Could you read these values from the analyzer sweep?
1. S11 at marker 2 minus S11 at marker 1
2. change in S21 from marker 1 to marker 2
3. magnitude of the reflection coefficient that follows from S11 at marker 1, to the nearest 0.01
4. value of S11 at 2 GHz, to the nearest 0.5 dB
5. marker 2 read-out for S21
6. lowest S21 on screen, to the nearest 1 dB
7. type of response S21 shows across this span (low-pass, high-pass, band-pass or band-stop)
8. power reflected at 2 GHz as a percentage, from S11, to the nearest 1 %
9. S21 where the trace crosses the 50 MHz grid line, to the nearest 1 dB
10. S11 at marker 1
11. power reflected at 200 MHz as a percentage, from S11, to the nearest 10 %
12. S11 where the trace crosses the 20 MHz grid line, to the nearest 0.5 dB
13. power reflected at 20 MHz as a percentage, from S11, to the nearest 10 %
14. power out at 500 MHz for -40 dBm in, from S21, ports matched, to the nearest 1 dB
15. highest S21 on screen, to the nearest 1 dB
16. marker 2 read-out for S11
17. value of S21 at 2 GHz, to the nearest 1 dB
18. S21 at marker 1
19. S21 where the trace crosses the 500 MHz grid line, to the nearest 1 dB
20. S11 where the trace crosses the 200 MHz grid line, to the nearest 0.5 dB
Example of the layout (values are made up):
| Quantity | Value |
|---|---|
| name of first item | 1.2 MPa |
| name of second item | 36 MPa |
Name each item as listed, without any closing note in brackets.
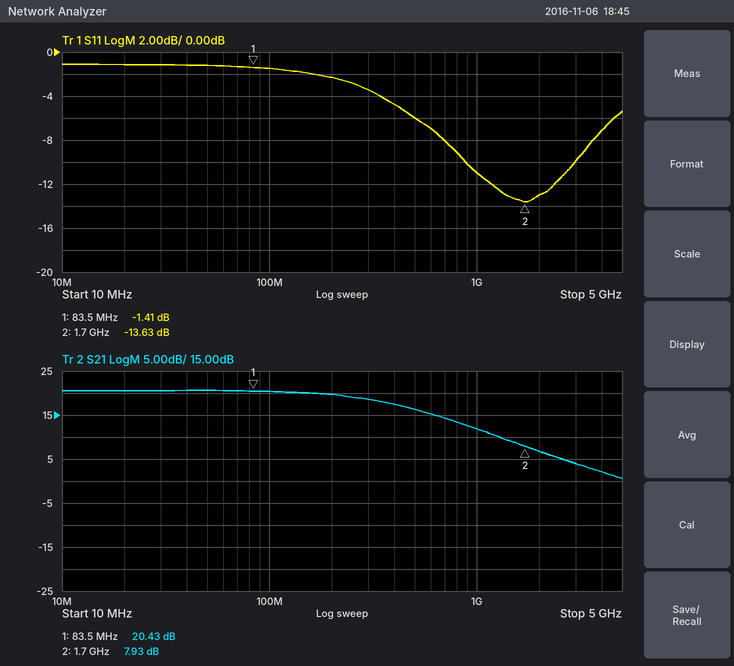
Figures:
| Quantity | Value |
|---|---|
| S11 at marker 2 minus S11 at marker 1 | -12.22 dB |
| change in S21 from marker 1 to marker 2 | -12.50 dB |
| magnitude of the reflection coefficient that follows from S11 at marker 1, to the nearest 0.01 | 0.85 |
| value of S11 at 2 GHz, to the nearest 0.5 dB | -13.0 dB |
| marker 2 read-out for S21 | 7.93 dB |
| lowest S21 on screen, to the nearest 1 dB | 1 dB |
| type of response S21 shows across this span | low-pass |
| power reflected at 2 GHz as a percentage, from S11, to the nearest 1 % | 5 % |
| S21 where the trace crosses the 50 MHz grid line, to the nearest 1 dB | 21 dB |
| S11 at marker 1 | -1.41 dB |
| power reflected at 200 MHz as a percentage, from S11, to the nearest 10 % | 60 % |
| S11 where the trace crosses the 20 MHz grid line, to the nearest 0.5 dB | -1.0 dB |
| power reflected at 20 MHz as a percentage, from S11, to the nearest 10 % | 80 % |
| power out at 500 MHz for -40 dBm in, from S21, ports matched, to the nearest 1 dB | -24 dBm |
| highest S21 on screen, to the nearest 1 dB | 21 dB |
| marker 2 read-out for S11 | -13.63 dB |
| value of S21 at 2 GHz, to the nearest 1 dB | 7 dB |
| S21 at marker 1 | 20.43 dB |
| S21 where the trace crosses the 500 MHz grid line, to the nearest 1 dB | 16 dB |
| S11 where the trace crosses the 200 MHz grid line, to the nearest 0.5 dB | -2.5 dB |
